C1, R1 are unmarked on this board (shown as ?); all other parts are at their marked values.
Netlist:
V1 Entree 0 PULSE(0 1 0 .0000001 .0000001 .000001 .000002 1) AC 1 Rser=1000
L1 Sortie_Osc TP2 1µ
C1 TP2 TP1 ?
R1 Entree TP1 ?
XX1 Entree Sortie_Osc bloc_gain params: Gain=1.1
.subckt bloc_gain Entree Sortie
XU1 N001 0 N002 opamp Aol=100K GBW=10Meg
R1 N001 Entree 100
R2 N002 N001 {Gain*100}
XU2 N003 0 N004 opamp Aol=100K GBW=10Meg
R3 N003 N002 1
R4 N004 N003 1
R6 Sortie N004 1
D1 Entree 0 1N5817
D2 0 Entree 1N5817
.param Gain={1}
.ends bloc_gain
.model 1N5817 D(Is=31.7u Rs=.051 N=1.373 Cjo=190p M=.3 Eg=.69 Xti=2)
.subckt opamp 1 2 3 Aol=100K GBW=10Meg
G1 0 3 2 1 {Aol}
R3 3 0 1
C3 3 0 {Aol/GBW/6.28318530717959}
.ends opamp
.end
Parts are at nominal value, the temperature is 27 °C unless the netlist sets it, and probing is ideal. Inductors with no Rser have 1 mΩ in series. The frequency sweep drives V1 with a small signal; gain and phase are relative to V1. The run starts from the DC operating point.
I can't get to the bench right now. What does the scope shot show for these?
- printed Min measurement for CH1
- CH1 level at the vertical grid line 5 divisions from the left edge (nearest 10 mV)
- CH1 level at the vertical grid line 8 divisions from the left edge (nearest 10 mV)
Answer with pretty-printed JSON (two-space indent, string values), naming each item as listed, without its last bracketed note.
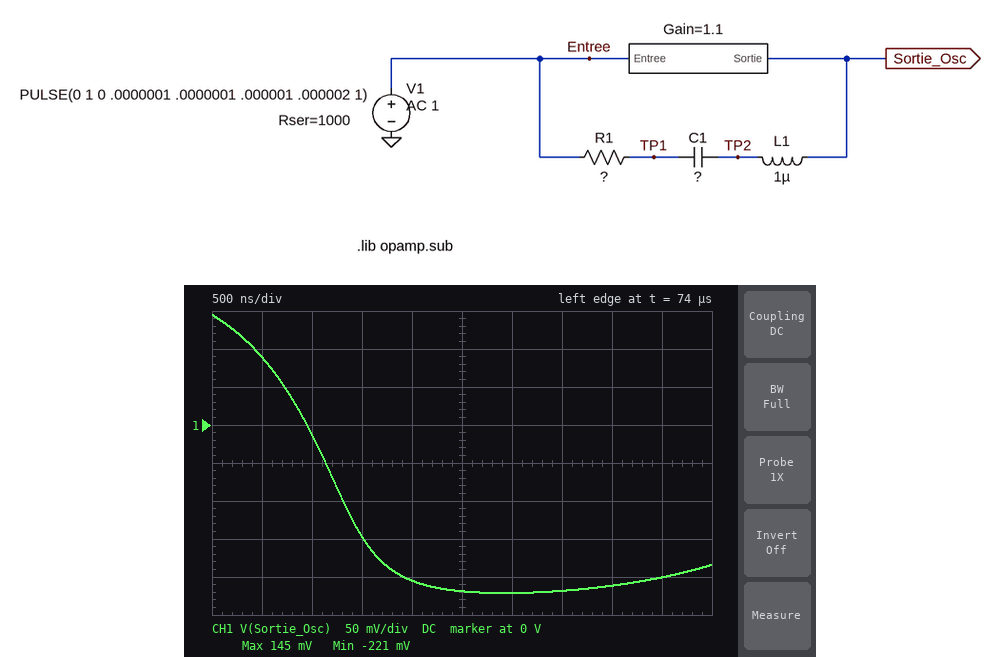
{
  "printed Min measurement for CH1": "-221 mV",
  "CH1 level at the vertical grid line 5 divisions from the left edge": "-220 mV",
  "CH1 level at the vertical grid line 8 divisions from the left edge": "-210 mV"
}
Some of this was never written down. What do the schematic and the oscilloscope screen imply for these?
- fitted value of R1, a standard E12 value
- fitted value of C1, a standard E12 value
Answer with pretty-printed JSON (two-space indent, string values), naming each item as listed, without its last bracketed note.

{
  "fitted value of R1, a standard E12 value": "0.68 Ω",
  "fitted value of C1, a standard E12 value": "1.2 µF"
}
